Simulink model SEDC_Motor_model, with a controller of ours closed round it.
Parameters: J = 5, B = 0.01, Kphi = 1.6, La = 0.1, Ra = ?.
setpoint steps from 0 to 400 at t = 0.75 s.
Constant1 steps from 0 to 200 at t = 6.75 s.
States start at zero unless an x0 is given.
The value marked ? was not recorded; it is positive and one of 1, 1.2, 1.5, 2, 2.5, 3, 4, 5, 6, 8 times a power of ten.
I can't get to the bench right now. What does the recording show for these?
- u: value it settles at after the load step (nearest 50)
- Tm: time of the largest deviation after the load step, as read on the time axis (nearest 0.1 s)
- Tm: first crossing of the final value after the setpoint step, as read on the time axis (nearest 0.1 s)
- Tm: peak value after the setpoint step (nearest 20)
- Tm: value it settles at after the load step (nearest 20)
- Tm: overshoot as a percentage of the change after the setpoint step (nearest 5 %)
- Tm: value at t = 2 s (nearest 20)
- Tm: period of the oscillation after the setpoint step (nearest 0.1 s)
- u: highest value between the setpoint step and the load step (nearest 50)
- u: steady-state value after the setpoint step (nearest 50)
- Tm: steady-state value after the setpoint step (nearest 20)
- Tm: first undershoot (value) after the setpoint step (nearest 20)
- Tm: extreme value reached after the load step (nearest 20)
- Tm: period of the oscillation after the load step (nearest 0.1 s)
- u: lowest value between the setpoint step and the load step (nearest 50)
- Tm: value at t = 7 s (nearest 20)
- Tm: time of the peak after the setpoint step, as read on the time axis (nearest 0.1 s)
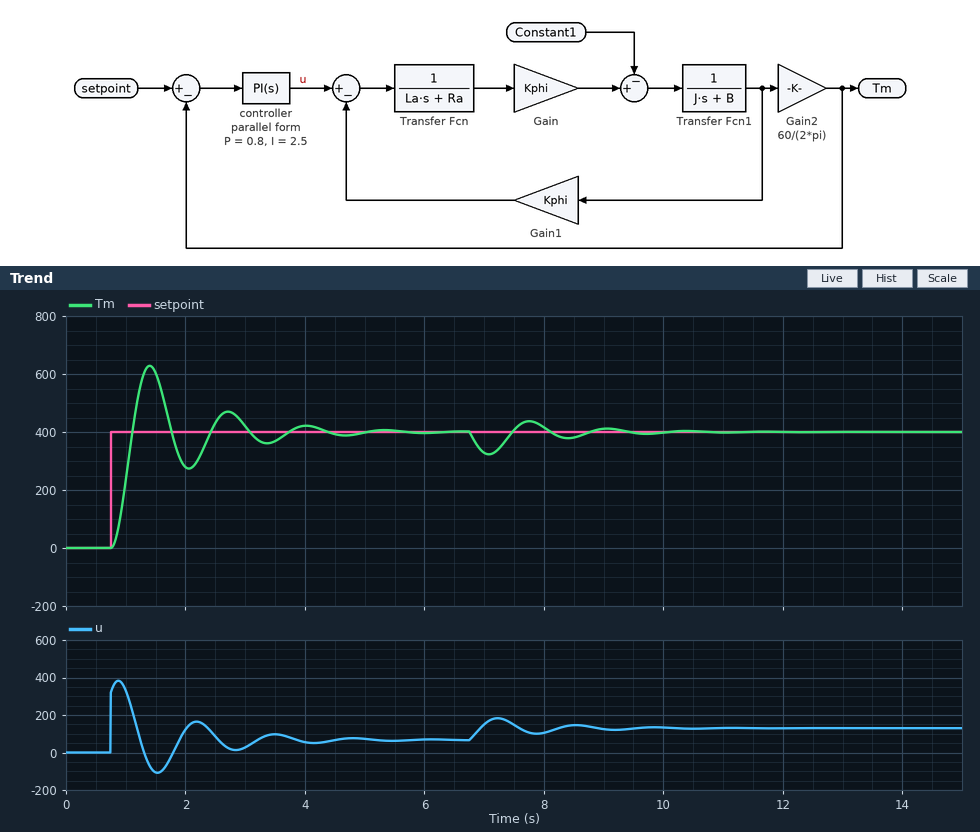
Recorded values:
150
7.1 s
1.1 s
620
400
55 %
280
1.3 s
400
50
400
280
320
1.3 s
-100
320
1.4 s
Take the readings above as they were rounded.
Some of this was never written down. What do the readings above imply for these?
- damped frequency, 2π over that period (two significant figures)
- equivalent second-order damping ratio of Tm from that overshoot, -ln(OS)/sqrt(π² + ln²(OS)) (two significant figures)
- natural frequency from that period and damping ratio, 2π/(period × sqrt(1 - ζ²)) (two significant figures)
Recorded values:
4.8 rad/s
0.19
4.9 rad/s
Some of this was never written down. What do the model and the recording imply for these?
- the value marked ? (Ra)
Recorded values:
0.5
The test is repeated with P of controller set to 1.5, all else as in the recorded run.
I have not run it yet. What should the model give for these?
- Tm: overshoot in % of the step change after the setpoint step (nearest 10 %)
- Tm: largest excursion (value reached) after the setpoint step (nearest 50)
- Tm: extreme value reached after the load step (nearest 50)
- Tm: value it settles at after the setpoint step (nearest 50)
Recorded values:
50 %
600
350
400
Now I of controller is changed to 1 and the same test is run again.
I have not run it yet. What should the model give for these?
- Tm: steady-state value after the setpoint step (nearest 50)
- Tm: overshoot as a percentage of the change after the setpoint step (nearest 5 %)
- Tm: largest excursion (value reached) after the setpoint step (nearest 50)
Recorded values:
400
25 %
500
